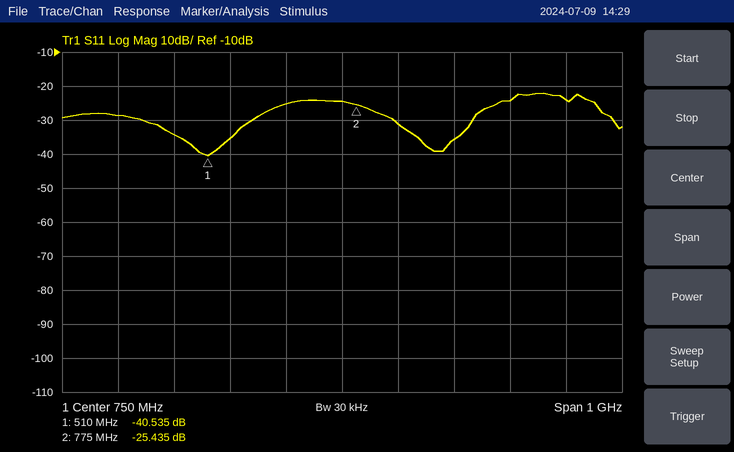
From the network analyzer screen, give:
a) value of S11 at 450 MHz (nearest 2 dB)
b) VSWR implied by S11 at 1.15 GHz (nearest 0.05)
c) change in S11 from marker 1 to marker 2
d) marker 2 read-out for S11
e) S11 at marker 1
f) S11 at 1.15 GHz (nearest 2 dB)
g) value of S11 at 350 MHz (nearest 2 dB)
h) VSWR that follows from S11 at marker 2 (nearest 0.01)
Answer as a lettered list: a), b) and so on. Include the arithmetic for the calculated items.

a) -34 dB
b) |Γ| = 10^(-24/20) = 0.0631; VSWR = (1 + 0.0631)/(1 − 0.0631) ≈ 1.13, so 1.15 to the nearest 0.05
c) -25.435 − (-40.535) = 15.100 dB
d) -25.435 dB
e) -40.535 dB
f) -24 dB
g) -28 dB
h) (1 + 0.0535)/(1 − 0.0535) ≈ 1.11
